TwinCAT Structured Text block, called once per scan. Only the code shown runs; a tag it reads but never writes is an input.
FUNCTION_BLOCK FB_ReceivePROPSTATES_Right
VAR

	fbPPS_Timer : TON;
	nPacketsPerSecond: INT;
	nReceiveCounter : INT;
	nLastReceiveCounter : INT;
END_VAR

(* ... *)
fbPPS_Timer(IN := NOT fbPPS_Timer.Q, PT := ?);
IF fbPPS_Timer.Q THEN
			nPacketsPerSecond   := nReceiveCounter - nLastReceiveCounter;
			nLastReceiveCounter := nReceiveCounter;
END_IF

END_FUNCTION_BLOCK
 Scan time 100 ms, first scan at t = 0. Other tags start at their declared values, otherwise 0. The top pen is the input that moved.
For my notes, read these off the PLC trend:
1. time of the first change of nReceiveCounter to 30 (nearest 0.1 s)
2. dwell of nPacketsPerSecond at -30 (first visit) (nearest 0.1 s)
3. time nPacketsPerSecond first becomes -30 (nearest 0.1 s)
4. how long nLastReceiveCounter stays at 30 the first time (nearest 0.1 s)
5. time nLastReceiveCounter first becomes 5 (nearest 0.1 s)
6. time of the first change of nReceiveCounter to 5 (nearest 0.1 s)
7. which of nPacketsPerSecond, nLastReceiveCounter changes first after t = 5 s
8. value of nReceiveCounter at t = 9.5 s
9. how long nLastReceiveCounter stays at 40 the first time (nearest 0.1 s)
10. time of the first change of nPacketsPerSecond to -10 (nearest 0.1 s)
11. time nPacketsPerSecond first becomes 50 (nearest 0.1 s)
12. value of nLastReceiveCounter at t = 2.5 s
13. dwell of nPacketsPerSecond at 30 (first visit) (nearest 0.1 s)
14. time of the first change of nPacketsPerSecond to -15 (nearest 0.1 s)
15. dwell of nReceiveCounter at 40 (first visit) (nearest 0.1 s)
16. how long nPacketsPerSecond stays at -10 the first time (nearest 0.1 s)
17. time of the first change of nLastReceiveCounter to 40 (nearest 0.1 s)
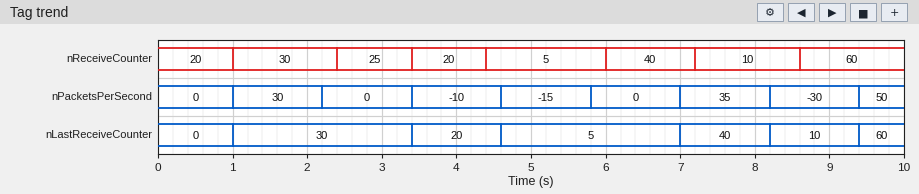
1.0 s
1.2 s
8.2 s
2.4 s
4.6 s
4.4 s
nPacketsPerSecond
60
1.2 s
3.4 s
9.4 s
30
1.2 s
4.6 s
1.2 s
1.2 s
7.0 s
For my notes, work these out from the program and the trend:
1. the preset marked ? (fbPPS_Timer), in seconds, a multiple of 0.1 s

1.0 s
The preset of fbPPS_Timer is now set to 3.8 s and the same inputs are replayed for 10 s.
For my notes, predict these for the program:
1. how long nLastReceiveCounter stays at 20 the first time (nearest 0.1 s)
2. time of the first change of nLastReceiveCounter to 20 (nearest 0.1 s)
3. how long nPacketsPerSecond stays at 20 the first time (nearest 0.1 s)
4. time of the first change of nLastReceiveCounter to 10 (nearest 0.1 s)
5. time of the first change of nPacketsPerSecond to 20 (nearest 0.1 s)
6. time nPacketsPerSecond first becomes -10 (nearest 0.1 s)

4.0 s
3.8 s
4.0 s
7.8 s
3.8 s
7.8 s
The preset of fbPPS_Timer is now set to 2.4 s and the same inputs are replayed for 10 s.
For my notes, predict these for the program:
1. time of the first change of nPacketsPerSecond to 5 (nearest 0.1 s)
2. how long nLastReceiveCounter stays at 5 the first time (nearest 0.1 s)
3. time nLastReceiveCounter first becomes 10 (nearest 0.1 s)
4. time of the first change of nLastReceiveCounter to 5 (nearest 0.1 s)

7.6 s
2.6 s
7.6 s
5.0 s
